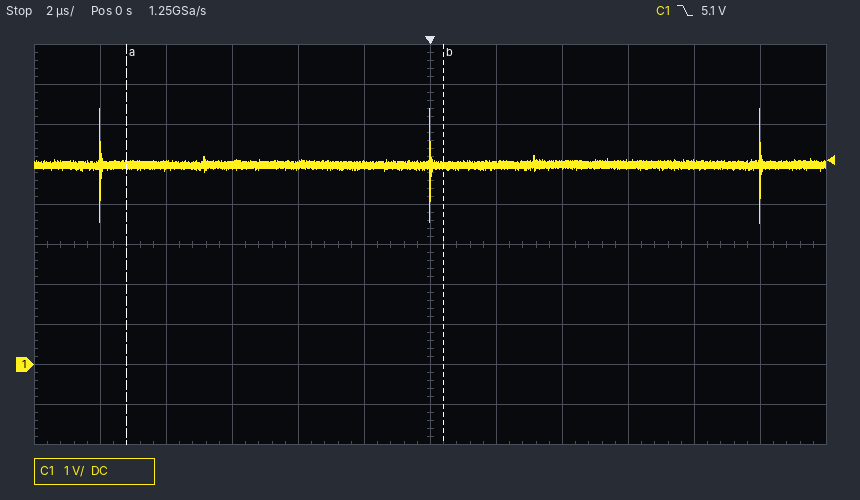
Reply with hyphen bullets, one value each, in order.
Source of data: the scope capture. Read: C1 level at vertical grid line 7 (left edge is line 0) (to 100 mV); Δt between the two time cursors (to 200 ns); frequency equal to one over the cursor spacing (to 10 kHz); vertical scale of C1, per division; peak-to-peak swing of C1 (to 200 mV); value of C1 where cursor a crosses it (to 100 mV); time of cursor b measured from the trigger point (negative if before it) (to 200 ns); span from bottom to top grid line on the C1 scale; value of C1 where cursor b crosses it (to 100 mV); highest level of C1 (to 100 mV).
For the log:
- 5.0 V
- 9.6 µs
- 100 kHz
- 1 V
- 2.8 V
- 5.0 V
- +400 ns
- 10 V
- 5.0 V
- 6.4 V
